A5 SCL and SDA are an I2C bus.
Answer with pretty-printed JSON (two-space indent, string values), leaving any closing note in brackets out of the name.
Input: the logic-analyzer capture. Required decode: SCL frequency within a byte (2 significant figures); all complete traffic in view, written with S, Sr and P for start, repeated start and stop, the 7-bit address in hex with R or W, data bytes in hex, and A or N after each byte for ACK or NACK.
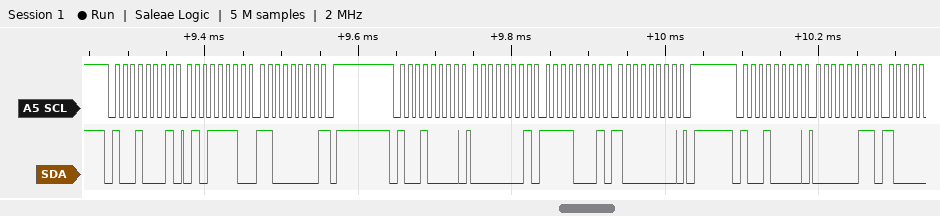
{
  "SCL frequency within a byte": "100 kHz",
  "all complete traffic in view, written with S, Sr and P for start, repeated start and stop, the 7-bit address in hex with R or W, data bytes in hex, and A or N after each byte for ACK or NACK": "S 48R A 5E A C0 N P S 48W A 01 A F1 A 80 A P S 48W A 03 A"
}
